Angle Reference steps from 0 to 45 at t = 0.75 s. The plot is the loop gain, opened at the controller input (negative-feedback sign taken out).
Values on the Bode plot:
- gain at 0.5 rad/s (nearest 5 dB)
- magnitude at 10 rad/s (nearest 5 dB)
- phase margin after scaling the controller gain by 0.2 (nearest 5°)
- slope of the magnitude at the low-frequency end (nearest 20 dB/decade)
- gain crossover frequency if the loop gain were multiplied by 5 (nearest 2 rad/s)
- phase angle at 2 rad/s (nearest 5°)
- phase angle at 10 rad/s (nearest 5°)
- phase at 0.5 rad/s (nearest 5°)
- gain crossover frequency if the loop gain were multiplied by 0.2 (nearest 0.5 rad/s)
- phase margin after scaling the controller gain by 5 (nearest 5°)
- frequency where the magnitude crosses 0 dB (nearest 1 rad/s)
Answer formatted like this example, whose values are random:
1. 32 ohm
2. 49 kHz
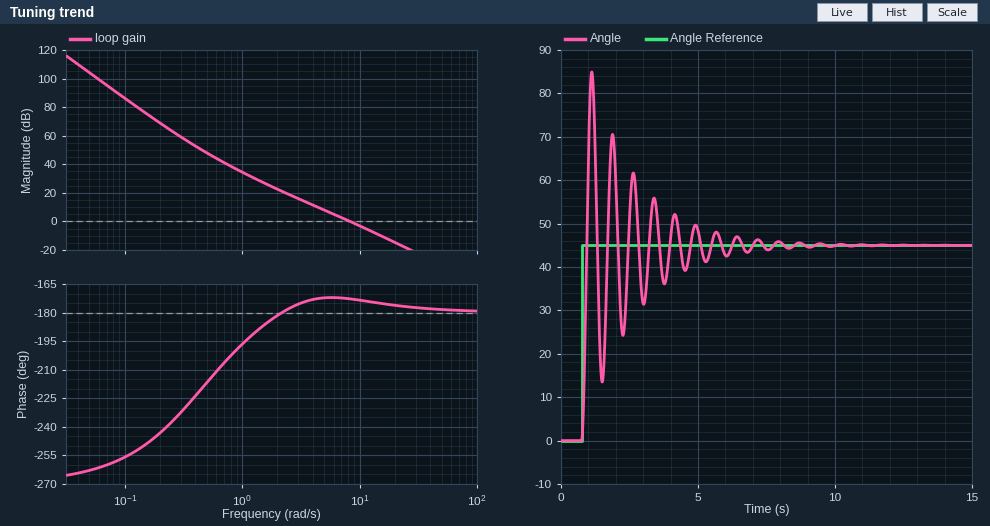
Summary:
1. 50 dB
2. -5 dB
3. 5°
4. -60 dB/decade
5. 20 rad/s
6. -180°
7. -175°
8. -215°
9. 3.5 rad/s
10. 5°
11. 8 rad/s
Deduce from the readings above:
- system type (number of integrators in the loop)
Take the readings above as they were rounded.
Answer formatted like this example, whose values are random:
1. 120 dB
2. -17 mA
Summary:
1. 3
